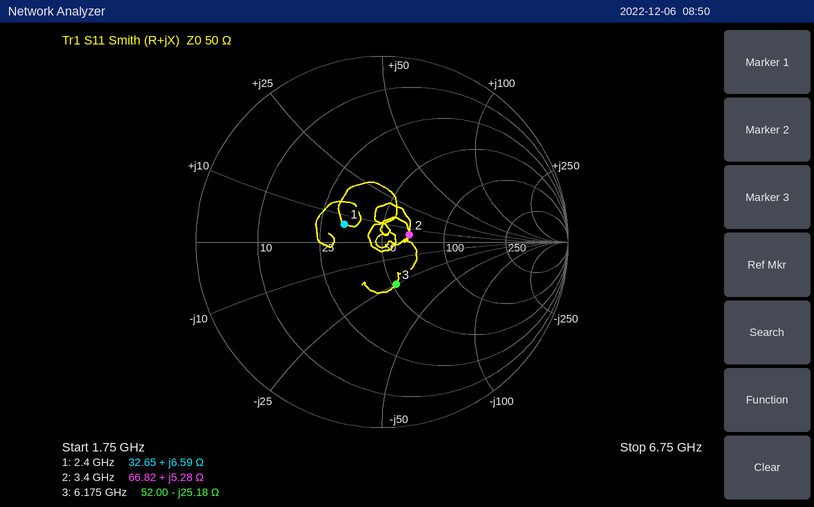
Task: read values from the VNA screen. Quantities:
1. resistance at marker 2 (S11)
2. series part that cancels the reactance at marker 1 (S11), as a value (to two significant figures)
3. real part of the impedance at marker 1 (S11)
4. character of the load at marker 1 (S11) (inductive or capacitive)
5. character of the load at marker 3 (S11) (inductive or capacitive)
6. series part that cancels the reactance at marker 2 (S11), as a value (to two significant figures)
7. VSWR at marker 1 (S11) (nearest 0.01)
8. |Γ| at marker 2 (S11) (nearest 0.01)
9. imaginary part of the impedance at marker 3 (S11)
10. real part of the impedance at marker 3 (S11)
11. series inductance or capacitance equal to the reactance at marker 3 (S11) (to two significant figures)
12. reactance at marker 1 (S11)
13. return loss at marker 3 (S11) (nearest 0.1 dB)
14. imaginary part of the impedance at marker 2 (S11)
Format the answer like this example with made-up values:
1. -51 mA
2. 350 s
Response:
1. 66.82 Ω
2. 10 pF
3. 32.65 Ω
4. inductive
5. capacitive
6. 8.9 pF
7. 1.58
8. 0.15
9. -25.18 Ω
10. 52.00 Ω
11. 1.0 pF
12. +6.59 Ω
13. 12.4 dB
14. +5.28 Ω
